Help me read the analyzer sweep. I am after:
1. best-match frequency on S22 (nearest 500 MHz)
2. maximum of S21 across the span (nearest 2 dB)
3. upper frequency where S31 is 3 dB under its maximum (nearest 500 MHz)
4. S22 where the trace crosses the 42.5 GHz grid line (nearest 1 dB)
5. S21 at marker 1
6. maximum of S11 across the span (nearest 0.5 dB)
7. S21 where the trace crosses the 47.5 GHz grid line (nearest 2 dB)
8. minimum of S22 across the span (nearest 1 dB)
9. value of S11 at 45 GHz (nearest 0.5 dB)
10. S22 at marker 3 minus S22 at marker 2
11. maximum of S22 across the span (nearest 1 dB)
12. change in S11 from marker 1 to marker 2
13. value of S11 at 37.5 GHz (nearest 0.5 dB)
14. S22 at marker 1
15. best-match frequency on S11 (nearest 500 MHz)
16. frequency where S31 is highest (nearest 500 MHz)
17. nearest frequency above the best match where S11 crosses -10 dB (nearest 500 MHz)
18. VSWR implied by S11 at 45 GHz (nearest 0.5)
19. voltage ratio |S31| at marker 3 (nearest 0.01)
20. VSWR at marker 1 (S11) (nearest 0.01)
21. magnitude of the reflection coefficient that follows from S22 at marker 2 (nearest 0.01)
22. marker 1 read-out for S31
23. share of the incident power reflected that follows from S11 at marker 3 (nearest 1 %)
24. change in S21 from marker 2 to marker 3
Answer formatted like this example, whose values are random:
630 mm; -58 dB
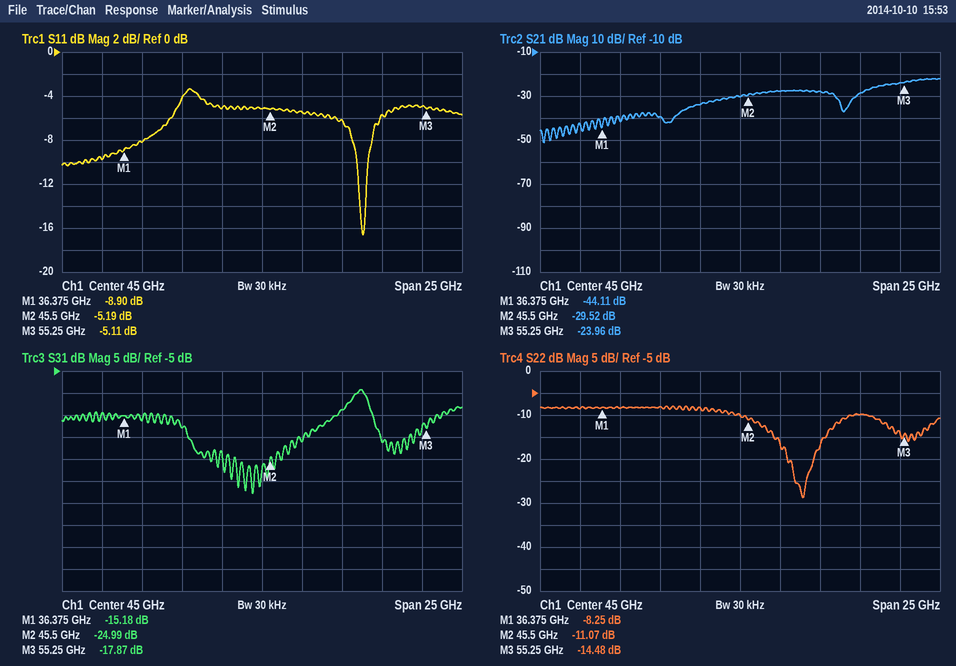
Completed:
49.0 GHz; -22 dB; 51.5 GHz; -8 dB; -44.11 dB; -3.5 dB; -28 dB; -29 dB; -5.0 dB; -3.41 dB; -8 dB; 3.71 dB; -8.0 dB; -8.25 dB; 51.5 GHz; 51.0 GHz; 51.5 GHz; 3.5; 0.13; 2.12; 0.28; -15.18 dB; 31 %; 5.56 dB
